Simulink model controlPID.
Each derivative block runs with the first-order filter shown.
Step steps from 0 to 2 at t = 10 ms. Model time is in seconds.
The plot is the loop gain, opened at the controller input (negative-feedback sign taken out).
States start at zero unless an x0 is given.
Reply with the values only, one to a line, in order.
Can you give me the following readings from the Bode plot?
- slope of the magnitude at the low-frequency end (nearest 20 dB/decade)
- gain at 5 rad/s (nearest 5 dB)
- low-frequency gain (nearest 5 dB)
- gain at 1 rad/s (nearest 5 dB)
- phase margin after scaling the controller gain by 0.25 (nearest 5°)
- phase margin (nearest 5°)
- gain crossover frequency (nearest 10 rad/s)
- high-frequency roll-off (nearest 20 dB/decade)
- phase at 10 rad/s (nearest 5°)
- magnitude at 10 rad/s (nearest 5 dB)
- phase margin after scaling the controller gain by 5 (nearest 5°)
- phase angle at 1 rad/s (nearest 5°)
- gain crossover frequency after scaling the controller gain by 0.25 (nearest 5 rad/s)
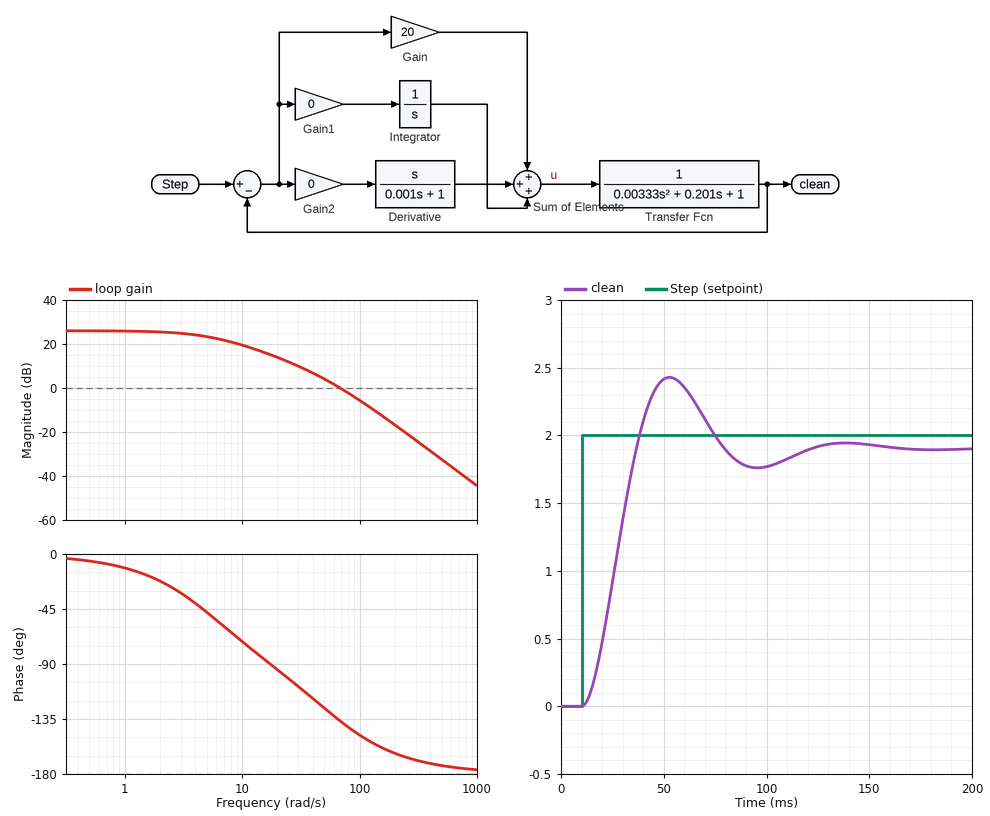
0 dB/decade
25 dB
25 dB
25 dB
80°
45°
70 rad/s
-40 dB/decade
-70°
20 dB
20°
-10°
25 rad/s
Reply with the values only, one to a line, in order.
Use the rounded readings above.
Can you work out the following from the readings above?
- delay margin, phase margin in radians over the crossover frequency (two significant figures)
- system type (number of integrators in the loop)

0.011 s
0
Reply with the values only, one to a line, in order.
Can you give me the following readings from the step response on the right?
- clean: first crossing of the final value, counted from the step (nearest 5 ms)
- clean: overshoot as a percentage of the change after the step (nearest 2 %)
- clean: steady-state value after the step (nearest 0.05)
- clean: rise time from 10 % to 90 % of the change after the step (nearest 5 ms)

25 ms
28 %
1.90
20 ms
